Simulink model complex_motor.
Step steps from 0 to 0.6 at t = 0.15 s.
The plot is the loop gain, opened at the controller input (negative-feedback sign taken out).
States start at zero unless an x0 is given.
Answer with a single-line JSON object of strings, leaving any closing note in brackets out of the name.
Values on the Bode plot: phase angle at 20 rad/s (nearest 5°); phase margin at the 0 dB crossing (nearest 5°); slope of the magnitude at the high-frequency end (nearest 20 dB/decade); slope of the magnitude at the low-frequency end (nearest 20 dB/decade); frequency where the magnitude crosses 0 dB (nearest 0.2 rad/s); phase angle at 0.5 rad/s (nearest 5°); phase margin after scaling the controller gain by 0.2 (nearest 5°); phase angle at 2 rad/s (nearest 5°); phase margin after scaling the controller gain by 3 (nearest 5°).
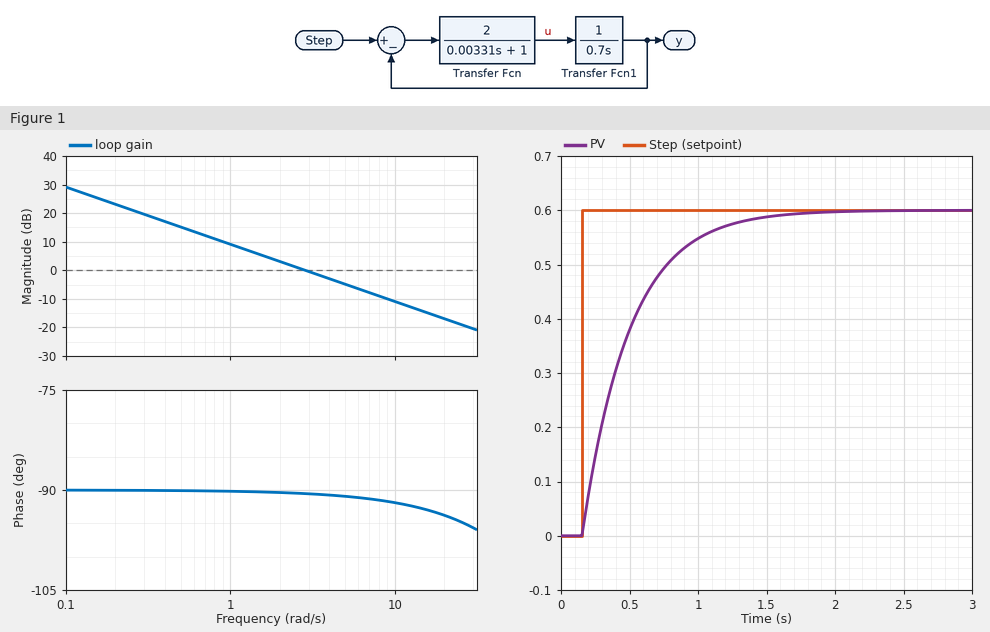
{"phase angle at 20 rad/s": "-95°", "phase margin at the 0 dB crossing": "90°", "slope of the magnitude at the high-frequency end": "-20 dB/decade", "slope of the magnitude at the low-frequency end": "-20 dB/decade", "frequency where the magnitude crosses 0 dB": "2.8 rad/s", "phase angle at 0.5 rad/s": "-90°", "phase margin after scaling the controller gain by 0.2": "90°", "phase angle at 2 rad/s": "-90°", "phase margin after scaling the controller gain by 3": "90°"}
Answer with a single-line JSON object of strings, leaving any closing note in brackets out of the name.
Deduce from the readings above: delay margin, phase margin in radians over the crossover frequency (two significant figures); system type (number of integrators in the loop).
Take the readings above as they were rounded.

{"delay margin, phase margin in radians over the crossover frequency": "0.56 s", "system type": "1"}
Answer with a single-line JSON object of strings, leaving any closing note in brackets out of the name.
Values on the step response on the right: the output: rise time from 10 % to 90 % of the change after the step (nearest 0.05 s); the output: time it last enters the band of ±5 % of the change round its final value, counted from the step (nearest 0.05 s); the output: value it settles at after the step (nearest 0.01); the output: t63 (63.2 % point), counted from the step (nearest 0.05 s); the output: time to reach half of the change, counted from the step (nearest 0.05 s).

{"the output: rise time from 10 % to 90 % of the change after the step": "0.75 s", "the output: time it last enters the band of ±5 % of the change round its final value, counted from the step": "1.05 s", "the output: value it settles at after the step": "0.60", "the output: t63 (63.2 % point), counted from the step": "0.35 s", "the output: time to reach half of the change, counted from the step": "0.25 s"}
